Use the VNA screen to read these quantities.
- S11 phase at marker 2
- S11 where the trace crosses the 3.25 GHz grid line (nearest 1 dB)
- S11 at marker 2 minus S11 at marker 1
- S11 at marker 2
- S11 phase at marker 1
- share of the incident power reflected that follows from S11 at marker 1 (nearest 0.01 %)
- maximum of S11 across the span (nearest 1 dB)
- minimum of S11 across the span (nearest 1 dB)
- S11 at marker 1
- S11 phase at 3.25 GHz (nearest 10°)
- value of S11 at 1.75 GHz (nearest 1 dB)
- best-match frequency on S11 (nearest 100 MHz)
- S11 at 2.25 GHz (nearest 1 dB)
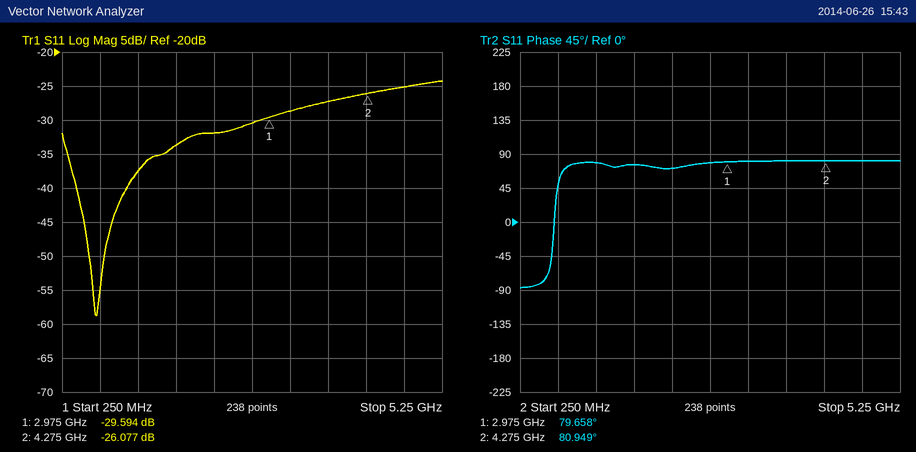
80.949°
-29 dB
3.517 dB
-26.077 dB
79.658°
0.11 %
-24 dB
-59 dB
-29.594 dB
80°
-34 dB
700 MHz
-32 dB
